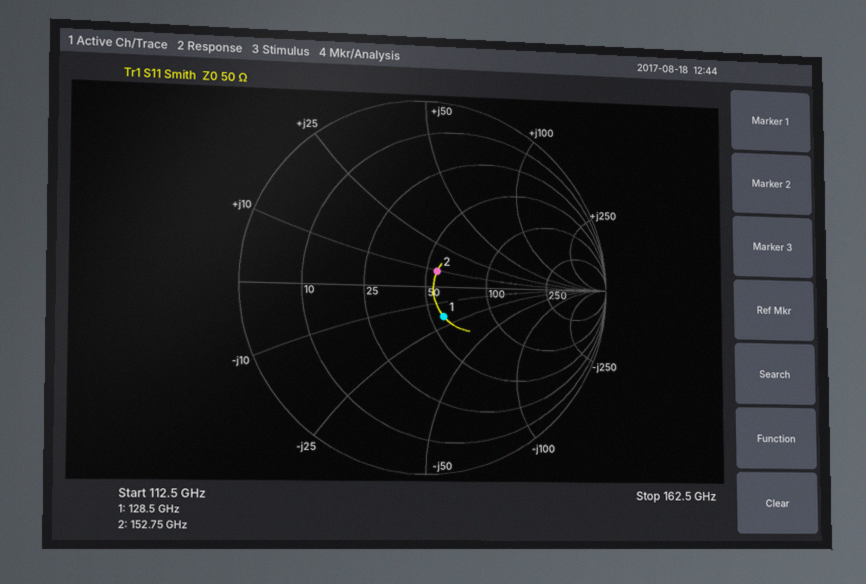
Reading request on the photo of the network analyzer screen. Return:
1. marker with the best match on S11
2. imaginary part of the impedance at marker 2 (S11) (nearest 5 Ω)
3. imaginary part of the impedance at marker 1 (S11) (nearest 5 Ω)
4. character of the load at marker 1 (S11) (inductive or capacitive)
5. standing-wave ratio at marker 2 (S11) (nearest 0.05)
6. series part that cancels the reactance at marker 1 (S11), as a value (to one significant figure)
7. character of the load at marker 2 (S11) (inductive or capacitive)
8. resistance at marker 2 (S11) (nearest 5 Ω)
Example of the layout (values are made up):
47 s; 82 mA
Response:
marker 2; +10 Ω; -20 Ω; capacitive; 1.25; 20 pH; inductive; 55 Ω
